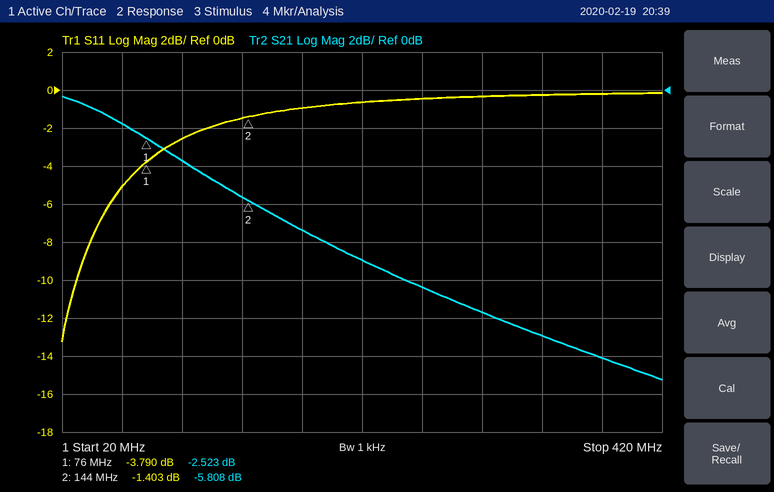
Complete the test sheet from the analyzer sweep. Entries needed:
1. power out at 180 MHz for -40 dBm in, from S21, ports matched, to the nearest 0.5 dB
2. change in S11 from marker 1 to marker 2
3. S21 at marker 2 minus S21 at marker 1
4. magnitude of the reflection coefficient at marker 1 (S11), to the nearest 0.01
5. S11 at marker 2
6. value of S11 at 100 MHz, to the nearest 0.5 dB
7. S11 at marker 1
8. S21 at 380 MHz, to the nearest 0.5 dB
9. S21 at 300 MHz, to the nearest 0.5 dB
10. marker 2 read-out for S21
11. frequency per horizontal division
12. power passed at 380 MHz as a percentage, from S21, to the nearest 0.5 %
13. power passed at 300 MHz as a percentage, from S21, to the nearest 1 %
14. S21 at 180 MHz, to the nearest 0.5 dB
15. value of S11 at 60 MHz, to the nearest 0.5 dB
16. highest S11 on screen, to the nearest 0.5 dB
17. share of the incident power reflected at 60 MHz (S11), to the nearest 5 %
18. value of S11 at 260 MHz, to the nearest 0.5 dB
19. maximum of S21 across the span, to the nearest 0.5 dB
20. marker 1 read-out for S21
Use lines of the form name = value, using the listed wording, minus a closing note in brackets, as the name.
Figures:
power out at 180 MHz for -40 dBm in, from S21, ports matched, to the nearest 0.5 dB = -47.5 dBm
change in S11 from marker 1 to marker 2 = 2.387 dB
S21 at marker 2 minus S21 at marker 1 = -3.285 dB
magnitude of the reflection coefficient at marker 1 (S11), to the nearest 0.01 = 0.65
S11 at marker 2 = -1.403 dB
value of S11 at 100 MHz, to the nearest 0.5 dB = -2.5 dB
S11 at marker 1 = -3.790 dB
S21 at 380 MHz, to the nearest 0.5 dB = -14.0 dB
S21 at 300 MHz, to the nearest 0.5 dB = -11.5 dB
marker 2 read-out for S21 = -5.808 dB
frequency per horizontal division = 40 MHz
power passed at 380 MHz as a percentage, from S21, to the nearest 0.5 % = 4.0 %
power passed at 300 MHz as a percentage, from S21, to the nearest 1 % = 7 %
S21 at 180 MHz, to the nearest 0.5 dB = -7.5 dB
value of S11 at 60 MHz, to the nearest 0.5 dB = -5.0 dB
highest S11 on screen, to the nearest 0.5 dB = 0.0 dB
share of the incident power reflected at 60 MHz (S11), to the nearest 5 % = 30 %
value of S11 at 260 MHz, to the nearest 0.5 dB = -0.5 dB
maximum of S21 across the span, to the nearest 0.5 dB = -0.5 dB
marker 1 read-out for S21 = -2.523 dB
